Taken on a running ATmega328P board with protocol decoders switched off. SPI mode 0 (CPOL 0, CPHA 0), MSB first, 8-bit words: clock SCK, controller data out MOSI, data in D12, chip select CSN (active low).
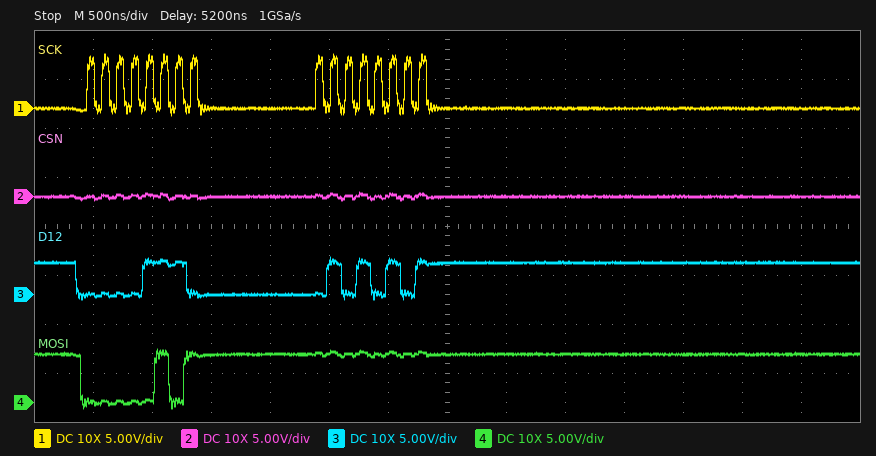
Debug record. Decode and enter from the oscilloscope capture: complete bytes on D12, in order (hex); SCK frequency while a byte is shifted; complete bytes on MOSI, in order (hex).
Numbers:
0E 55
8 MHz
05 FF
